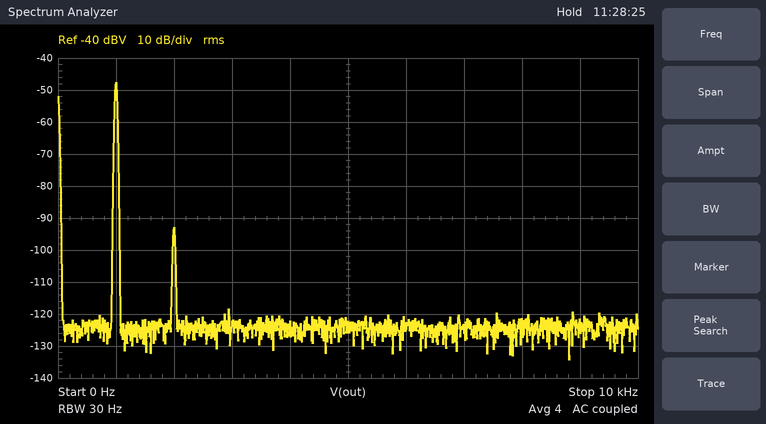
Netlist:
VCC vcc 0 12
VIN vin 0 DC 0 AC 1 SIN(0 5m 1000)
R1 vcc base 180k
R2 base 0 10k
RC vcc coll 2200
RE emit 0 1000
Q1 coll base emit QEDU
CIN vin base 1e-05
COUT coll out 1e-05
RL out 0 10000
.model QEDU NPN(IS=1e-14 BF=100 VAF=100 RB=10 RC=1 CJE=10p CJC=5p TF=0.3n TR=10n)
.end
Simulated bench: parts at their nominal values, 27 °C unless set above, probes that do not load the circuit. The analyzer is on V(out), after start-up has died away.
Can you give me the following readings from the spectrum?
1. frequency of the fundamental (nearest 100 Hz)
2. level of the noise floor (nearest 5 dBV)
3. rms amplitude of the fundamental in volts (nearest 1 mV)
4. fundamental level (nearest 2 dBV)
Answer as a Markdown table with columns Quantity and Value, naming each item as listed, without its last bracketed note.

| Quantity | Value |
|---|---|
| frequency of the fundamental | 1.0 kHz |
| level of the noise floor | -125 dBV |
| rms amplitude of the fundamental in volts | 4 mV |
| fundamental level | -48 dBV |
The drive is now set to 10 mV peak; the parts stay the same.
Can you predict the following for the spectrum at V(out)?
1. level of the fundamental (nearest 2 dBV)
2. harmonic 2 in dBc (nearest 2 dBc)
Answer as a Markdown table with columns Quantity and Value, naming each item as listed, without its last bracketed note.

| Quantity | Value |
|---|---|
| level of the fundamental | -42 dBV |
| harmonic 2 in dBc | -40 dBc |
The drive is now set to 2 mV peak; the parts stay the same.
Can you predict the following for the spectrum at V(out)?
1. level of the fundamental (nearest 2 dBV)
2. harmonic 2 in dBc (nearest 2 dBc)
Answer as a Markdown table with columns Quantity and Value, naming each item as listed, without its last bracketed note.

| Quantity | Value |
|---|---|
| level of the fundamental | -56 dBV |
| harmonic 2 in dBc | -54 dBc |
